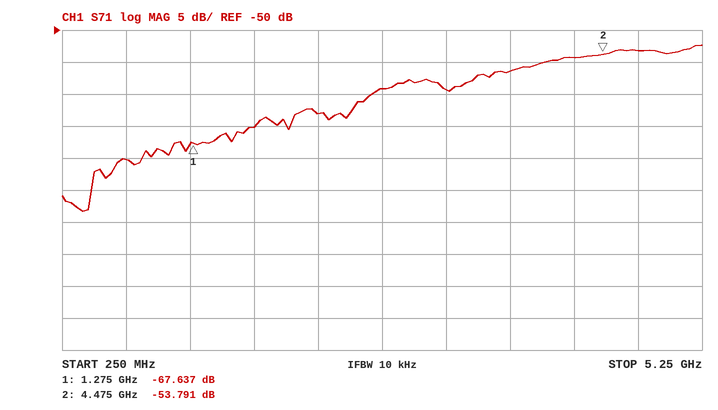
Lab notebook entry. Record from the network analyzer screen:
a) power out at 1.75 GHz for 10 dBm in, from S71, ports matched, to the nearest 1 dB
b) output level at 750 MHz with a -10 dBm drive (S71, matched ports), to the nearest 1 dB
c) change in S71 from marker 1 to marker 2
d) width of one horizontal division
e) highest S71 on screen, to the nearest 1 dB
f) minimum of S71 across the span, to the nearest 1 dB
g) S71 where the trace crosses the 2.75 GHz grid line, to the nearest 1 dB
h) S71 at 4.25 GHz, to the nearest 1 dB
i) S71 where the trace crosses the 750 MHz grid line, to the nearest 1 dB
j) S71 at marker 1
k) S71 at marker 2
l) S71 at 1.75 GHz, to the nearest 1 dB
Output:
-55 dBm
-80 dBm
13.846 dB
500 MHz
-52 dB
-78 dB
-59 dB
-54 dB
-70 dB
-67.637 dB
-53.791 dB
-65 dB
